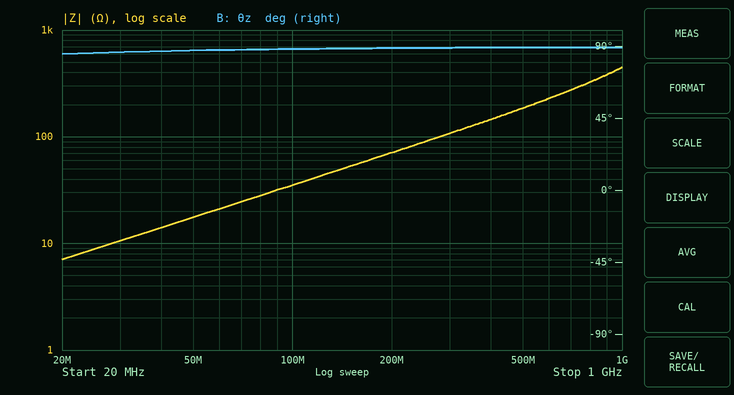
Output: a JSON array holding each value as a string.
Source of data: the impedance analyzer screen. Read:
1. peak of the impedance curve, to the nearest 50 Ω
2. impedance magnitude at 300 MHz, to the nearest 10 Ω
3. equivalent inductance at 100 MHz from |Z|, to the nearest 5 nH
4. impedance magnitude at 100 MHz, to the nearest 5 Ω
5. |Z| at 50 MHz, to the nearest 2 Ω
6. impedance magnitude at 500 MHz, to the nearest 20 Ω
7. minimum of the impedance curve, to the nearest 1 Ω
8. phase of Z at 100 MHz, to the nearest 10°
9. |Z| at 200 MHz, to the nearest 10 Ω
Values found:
["450 Ω", "110 Ω", "55 nH", "35 Ω", "18 Ω", "180 Ω", "7 Ω", "90°", "70 Ω"]
